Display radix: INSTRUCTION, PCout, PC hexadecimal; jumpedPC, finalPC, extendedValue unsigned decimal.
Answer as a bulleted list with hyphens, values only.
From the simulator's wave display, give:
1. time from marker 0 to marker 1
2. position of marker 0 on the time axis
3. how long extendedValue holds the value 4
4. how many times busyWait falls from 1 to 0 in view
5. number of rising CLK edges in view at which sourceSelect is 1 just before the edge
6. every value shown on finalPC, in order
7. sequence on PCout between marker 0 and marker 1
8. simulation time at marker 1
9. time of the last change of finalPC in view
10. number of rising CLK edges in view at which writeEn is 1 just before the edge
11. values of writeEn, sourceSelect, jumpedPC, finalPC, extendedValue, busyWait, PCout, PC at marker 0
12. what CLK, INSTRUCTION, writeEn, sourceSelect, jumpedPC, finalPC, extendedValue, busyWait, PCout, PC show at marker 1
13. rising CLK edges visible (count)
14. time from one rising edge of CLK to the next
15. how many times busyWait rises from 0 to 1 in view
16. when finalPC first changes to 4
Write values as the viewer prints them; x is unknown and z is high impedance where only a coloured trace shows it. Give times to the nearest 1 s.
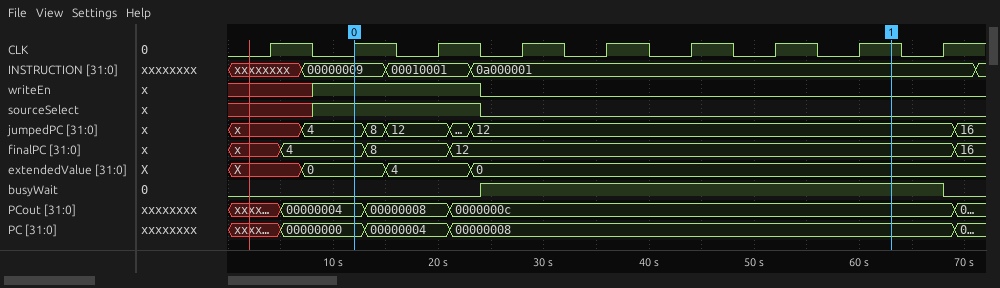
- 51 s
- 12 s
- 8 s
- 1
- 2
- x, 4, 8, 12, 16
- 00000004, 00000008, 0000000c
- 63 s
- 69 s
- 2
- writeEn=1, sourceSelect=1, jumpedPC=4, finalPC=4, extendedValue=0, busyWait=0, PCout=00000004, PC=00000000
- CLK=1, INSTRUCTION=0a000001, writeEn=0, sourceSelect=0, jumpedPC=12, finalPC=12, extendedValue=0, busyWait=1, PCout=0000000c, PC=00000008
- 9
- 8 s
- 1
- 5 s
